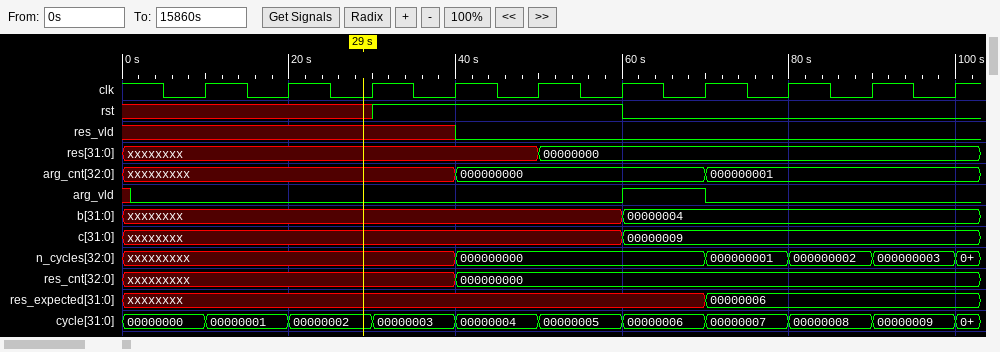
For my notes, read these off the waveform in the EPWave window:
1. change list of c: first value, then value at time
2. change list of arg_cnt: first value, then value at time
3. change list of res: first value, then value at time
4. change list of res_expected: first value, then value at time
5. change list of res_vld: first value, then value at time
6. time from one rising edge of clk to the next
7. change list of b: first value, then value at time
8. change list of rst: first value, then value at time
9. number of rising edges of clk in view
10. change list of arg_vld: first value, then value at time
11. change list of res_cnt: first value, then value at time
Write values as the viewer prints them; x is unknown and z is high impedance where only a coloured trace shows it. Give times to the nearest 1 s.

xxxxxxxx, 00000009 at 60 s
xxxxxxxxx, 000000000 at 40 s, 000000001 at 70 s
xxxxxxxx, 00000000 at 50 s
xxxxxxxx, 00000006 at 70 s
x, 0 at 40 s
10 s
xxxxxxxx, 00000004 at 60 s
x, 1 at 30 s, 0 at 60 s
10
x, 0 at 1 s, 1 at 60 s, 0 at 70 s
xxxxxxxxx, 000000000 at 40 s
